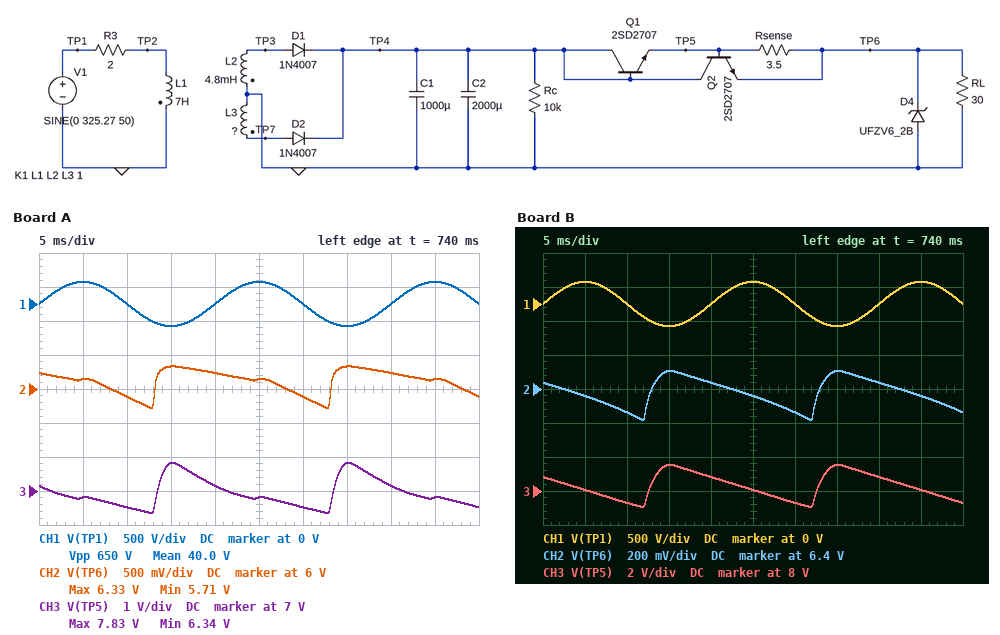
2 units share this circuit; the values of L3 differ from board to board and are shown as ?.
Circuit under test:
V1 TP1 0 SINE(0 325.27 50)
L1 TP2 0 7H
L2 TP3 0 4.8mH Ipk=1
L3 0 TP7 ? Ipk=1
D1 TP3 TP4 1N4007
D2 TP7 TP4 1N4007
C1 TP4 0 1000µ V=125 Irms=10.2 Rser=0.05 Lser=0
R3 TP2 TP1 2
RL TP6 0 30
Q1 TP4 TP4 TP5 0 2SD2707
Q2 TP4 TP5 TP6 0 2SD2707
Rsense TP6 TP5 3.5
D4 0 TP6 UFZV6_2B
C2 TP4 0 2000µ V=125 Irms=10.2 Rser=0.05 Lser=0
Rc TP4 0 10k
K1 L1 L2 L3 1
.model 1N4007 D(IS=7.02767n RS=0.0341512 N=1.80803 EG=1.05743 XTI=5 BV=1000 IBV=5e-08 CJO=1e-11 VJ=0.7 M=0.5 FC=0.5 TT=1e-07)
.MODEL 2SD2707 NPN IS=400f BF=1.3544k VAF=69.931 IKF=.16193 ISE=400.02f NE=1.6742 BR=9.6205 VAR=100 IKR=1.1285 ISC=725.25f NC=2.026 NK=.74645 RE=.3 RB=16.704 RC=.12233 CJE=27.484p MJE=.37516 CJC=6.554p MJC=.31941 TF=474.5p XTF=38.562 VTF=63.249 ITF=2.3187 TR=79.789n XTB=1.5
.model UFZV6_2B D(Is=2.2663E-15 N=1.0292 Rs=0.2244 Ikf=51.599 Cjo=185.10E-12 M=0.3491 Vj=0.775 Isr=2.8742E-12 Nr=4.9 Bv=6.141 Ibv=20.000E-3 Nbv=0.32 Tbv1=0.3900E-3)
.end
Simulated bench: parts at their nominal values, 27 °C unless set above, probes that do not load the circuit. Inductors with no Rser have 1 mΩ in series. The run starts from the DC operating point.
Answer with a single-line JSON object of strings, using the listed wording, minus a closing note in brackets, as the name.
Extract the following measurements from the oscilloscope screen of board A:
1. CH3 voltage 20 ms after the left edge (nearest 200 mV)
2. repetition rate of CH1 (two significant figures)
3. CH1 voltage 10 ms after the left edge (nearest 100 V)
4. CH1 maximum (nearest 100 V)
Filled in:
{"CH3 voltage 20 ms after the left edge": "7.2 V", "repetition rate of CH1": "50 Hz", "CH1 voltage 10 ms after the left edge": "0 V", "CH1 maximum": "300 V"}
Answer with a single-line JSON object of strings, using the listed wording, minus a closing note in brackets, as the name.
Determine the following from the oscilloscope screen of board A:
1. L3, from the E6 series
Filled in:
{"L3, from the E6 series": "6.8 mH"}
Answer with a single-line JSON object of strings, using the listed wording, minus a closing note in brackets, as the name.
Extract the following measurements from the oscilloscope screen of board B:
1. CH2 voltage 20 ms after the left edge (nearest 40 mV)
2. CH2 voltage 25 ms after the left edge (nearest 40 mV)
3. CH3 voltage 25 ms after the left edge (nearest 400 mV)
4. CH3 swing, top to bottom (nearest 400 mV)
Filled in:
{"CH2 voltage 20 ms after the left edge": "6.44 V", "CH2 voltage 25 ms after the left edge": "6.36 V", "CH3 voltage 25 ms after the left edge": "8.0 V", "CH3 swing, top to bottom": "2.4 V"}
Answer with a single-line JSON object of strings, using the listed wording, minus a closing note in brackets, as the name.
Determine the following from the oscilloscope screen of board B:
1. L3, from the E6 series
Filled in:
{"L3, from the E6 series": "15 mH"}
